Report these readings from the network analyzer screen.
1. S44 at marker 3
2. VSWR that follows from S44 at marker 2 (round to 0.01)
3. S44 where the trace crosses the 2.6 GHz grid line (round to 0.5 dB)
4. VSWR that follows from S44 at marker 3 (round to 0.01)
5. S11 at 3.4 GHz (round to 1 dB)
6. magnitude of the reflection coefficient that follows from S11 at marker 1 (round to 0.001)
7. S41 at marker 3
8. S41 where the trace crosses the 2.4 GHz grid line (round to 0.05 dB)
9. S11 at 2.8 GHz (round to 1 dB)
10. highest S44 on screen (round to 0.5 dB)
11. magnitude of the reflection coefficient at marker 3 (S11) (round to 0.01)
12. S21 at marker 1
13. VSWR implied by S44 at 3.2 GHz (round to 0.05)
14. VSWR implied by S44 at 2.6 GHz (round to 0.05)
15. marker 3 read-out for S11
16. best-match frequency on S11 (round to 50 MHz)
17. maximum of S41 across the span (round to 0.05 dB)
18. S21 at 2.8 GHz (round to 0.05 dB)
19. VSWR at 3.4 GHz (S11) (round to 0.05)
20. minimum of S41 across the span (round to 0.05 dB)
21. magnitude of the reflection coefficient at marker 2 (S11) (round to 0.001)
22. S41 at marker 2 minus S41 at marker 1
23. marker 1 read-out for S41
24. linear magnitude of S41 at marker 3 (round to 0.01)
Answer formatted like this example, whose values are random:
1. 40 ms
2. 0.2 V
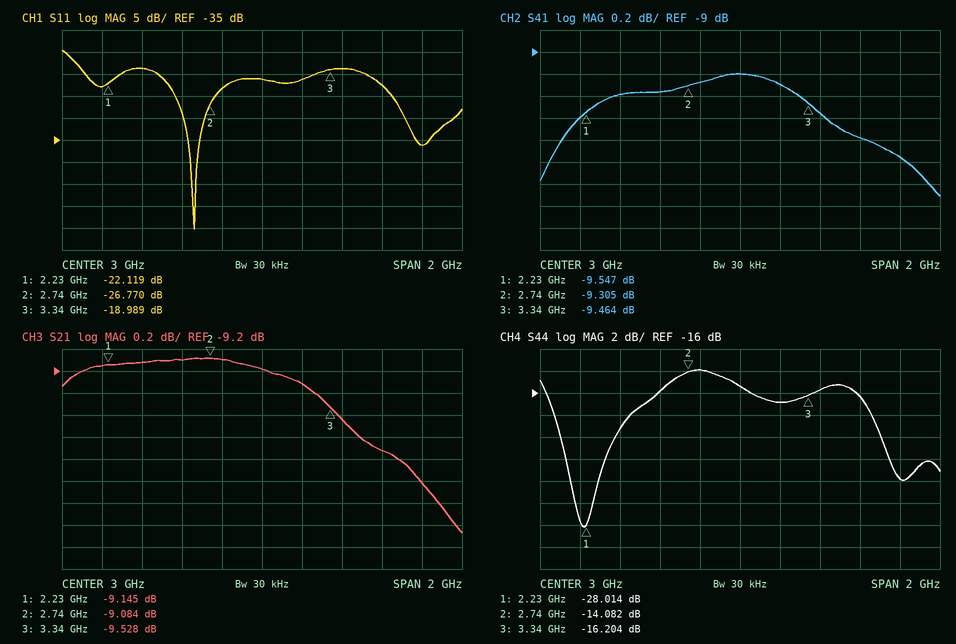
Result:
1. -16.204 dB
2. 1.49
3. -16.0 dB
4. 1.37
5. -19 dB
6. 0.078
7. -9.464 dB
8. -9.40 dB
9. -23 dB
10. -14.0 dB
11. 0.11
12. -9.145 dB
13. 1.35
14. 1.40
15. -18.989 dB
16. 2.65 GHz
17. -9.20 dB
18. -9.10 dB
19. 1.25
20. -10.30 dB
21. 0.046
22. 0.242 dB
23. -9.547 dB
24. 0.34
